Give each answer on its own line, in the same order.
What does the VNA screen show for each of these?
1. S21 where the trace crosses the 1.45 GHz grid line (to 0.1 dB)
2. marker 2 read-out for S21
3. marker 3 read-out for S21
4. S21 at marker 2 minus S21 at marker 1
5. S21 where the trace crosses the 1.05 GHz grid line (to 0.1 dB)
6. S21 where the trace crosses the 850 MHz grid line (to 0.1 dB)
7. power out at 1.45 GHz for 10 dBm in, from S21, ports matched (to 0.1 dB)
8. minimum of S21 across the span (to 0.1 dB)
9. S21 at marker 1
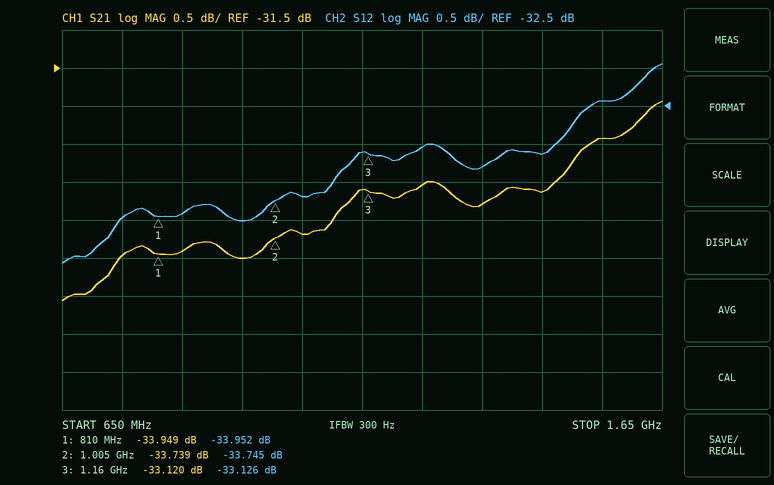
-33.1 dB
-33.739 dB
-33.120 dB
0.210 dB
-33.7 dB
-33.9 dB
-23.1 dBm
-34.6 dB
-33.949 dB
